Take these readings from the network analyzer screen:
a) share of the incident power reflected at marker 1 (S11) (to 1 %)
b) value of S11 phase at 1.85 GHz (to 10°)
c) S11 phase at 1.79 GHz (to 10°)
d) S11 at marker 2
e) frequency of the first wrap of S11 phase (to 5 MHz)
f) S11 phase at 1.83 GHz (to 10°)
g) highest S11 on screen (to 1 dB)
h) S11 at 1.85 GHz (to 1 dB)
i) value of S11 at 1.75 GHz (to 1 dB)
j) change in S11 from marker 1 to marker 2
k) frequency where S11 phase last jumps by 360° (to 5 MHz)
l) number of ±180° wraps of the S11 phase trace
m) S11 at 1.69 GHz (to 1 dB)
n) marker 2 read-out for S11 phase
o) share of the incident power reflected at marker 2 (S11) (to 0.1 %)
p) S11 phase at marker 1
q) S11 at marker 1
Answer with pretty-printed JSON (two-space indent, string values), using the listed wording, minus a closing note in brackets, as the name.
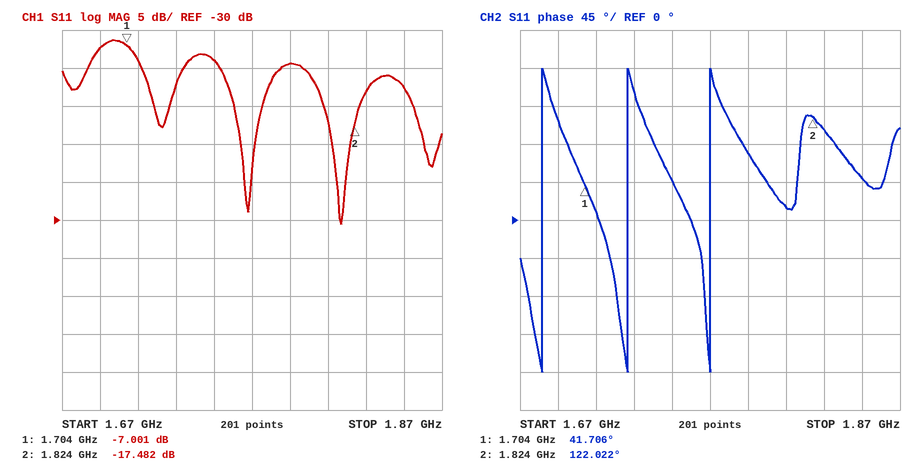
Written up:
{
  "share of the incident power reflected at marker 1 (S11)": "20 %",
  "value of S11 phase at 1.85 GHz": "50°",
  "S11 phase at 1.79 GHz": "80°",
  "S11 at marker 2": "-17.482 dB",
  "frequency of the first wrap of S11 phase": "1.680 GHz",
  "S11 phase at 1.83 GHz": "110°",
  "highest S11 on screen": "-6 dB",
  "S11 at 1.85 GHz": "-13 dB",
  "value of S11 at 1.75 GHz": "-9 dB",
  "change in S11 from marker 1 to marker 2": "-10.481 dB",
  "frequency where S11 phase last jumps by 360°": "1.770 GHz",
  "number of ±180° wraps of the S11 phase trace": "3",
  "S11 at 1.69 GHz": "-7 dB",
  "marker 2 read-out for S11 phase": "122.022°",
  "share of the incident power reflected at marker 2 (S11)": "1.8 %",
  "S11 phase at marker 1": "41.706°",
  "S11 at marker 1": "-7.001 dB"
}
